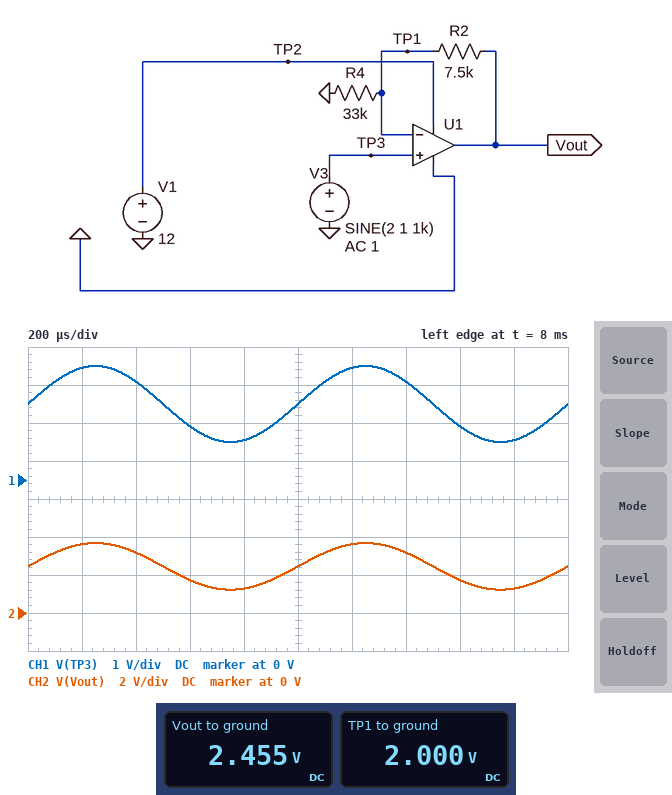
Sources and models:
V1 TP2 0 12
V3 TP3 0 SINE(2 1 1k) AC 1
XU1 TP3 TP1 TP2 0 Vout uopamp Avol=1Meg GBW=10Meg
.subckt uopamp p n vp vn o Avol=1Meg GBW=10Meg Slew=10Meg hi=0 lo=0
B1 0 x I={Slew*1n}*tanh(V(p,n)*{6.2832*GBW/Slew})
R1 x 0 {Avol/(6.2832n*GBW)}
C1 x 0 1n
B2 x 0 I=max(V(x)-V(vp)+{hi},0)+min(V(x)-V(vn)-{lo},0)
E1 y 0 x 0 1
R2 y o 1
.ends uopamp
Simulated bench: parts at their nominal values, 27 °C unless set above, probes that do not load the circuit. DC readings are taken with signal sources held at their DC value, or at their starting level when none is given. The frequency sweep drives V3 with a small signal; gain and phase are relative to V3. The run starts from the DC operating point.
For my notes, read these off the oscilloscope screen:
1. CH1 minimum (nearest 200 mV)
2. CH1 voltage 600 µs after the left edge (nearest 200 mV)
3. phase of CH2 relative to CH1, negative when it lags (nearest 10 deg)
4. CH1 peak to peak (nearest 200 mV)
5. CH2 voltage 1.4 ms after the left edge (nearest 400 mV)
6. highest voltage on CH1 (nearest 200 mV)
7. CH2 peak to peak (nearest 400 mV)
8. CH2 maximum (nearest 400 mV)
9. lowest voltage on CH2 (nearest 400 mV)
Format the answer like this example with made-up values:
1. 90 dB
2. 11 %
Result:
1. 1.0 V
2. 1.4 V
3. 0 deg
4. 2.0 V
5. 3.2 V
6. 3.0 V
7. 2.4 V
8. 3.6 V
9. 1.2 V
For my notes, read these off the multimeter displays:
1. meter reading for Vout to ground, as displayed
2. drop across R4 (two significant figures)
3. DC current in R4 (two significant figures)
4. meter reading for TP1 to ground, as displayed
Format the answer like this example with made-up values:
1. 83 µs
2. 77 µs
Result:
1. 2.455 V
2. 2.0 V
3. 61 µA
4. 2.000 V
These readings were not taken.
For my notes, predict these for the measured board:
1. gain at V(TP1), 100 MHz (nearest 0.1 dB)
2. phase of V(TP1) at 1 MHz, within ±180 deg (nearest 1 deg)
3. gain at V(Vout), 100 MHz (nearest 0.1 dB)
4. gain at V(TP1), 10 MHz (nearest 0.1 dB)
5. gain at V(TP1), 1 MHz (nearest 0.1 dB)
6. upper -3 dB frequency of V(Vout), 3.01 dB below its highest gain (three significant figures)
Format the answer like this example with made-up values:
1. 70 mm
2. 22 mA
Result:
1. -21.8 dB
2. -7 deg
3. -20.0 dB
4. -4.0 dB
5. -0.1 dB
6. 8.15 MHz
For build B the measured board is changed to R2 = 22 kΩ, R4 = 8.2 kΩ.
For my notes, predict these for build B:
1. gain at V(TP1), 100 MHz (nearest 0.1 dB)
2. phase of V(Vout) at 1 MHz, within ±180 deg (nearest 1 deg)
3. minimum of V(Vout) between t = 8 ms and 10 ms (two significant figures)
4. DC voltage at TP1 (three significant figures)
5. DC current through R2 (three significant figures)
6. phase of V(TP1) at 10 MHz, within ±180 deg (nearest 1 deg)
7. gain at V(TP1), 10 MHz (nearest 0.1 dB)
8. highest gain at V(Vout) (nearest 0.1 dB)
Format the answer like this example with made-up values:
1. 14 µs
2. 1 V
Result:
1. -31.3 dB
2. -20 deg
3. 3.7 V
4. 2.00 V
5. 244 µA
6. -75 deg
7. -11.6 dB
8. 11.3 dB
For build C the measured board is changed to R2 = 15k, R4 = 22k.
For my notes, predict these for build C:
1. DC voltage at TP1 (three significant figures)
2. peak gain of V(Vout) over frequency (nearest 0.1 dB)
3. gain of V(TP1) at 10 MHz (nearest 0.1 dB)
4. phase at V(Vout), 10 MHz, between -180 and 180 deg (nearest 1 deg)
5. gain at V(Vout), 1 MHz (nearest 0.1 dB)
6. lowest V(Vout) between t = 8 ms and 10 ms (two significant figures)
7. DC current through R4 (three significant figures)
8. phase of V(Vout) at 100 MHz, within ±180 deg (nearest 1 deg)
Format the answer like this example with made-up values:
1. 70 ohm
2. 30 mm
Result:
1. 2.00 V
2. 4.5 dB
3. -5.8 dB
4. -59 deg
5. 4.4 dB
6. 1.7 V
7. 90.9 µA
8. -87 deg
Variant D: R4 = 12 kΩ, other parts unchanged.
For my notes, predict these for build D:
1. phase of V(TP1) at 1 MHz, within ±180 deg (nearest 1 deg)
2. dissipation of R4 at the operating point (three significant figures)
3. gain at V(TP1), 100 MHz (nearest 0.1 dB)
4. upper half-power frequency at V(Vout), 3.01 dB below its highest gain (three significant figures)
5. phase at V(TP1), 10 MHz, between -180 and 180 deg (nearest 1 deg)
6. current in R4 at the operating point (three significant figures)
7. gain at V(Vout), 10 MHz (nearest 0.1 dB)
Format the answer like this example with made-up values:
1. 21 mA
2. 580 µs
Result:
1. -9 deg
2. 333 µW
3. -24.2 dB
4. 6.15 MHz
5. -58 deg
6. 167 µA
7. -1.4 dB
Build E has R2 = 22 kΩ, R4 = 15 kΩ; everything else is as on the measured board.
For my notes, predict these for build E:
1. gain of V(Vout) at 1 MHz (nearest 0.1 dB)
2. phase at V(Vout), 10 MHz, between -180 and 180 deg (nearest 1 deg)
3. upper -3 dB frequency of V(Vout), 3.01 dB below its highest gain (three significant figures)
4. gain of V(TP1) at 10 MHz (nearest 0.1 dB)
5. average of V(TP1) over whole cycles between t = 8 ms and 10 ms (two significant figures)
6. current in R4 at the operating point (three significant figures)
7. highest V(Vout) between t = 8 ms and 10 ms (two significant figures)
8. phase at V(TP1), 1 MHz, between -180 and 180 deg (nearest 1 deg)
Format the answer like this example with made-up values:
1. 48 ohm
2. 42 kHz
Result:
1. 7.6 dB
2. -68 deg
3. 4.05 MHz
4. -8.5 dB
5. 2.0 V
6. 133 µA
7. 7.4 V
8. -14 deg
